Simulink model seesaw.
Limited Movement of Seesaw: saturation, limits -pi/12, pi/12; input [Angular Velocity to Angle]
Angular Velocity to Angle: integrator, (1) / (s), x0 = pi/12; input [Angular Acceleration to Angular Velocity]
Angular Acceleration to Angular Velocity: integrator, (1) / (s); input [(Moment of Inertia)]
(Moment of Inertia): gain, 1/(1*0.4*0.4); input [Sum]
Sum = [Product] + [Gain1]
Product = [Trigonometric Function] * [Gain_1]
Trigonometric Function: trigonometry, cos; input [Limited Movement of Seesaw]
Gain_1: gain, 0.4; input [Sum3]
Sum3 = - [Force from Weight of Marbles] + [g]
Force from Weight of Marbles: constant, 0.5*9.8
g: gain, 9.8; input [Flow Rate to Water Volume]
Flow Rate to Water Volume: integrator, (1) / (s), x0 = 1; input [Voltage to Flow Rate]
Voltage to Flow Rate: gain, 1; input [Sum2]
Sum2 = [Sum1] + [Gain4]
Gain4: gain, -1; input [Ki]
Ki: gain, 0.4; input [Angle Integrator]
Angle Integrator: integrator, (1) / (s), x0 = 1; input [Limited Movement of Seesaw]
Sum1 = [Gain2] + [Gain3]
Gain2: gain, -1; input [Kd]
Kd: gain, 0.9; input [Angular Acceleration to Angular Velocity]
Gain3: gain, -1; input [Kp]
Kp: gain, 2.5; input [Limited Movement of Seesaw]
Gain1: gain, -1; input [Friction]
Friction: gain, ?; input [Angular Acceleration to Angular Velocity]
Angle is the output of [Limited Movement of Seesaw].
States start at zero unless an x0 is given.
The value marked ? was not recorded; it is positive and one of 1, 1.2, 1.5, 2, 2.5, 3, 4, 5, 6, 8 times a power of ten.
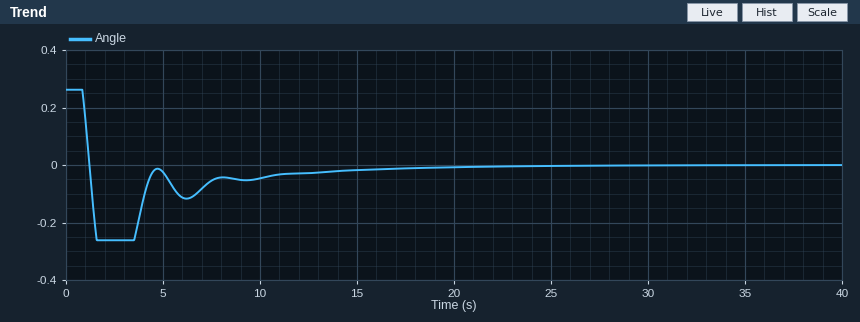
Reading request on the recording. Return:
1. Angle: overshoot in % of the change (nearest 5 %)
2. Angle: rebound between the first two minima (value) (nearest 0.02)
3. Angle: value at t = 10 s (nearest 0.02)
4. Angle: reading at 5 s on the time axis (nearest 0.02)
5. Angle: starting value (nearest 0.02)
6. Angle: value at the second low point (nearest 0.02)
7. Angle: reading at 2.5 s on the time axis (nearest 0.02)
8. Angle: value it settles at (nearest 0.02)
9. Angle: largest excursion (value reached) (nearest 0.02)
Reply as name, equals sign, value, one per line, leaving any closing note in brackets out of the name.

Angle: overshoot in % of the change = 100 %
Angle: rebound between the first two minima (value) = -0.02
Angle: value at t = 10 s = -0.04
Angle: reading at 5 s on the time axis = -0.02
Angle: starting value = 0.26
Angle: value at the second low point = -0.12
Angle: reading at 2.5 s on the time axis = -0.26
Angle: value it settles at = 0.00
Angle: largest excursion (value reached) = -0.26
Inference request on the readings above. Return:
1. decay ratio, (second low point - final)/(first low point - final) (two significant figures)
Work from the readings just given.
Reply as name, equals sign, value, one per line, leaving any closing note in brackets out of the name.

decay ratio, (second low point - final)/(first low point - final) = 0.46
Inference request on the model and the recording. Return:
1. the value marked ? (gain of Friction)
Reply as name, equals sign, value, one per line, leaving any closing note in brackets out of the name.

the value marked ? = 2.5
